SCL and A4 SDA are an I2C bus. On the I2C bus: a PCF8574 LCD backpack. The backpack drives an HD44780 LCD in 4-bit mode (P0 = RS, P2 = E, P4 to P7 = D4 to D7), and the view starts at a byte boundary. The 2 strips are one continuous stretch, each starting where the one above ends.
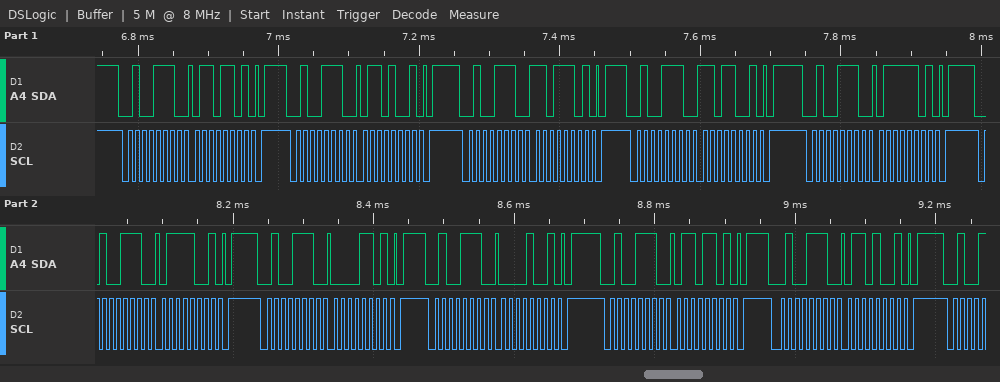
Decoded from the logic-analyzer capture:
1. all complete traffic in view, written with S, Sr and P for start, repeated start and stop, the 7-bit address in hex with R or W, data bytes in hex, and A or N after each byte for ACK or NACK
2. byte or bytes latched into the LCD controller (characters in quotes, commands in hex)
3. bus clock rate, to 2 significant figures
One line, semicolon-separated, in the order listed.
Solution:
S 27W A 6D A P S 27W A 69 A P S 27W A DD A P S 27W A D9 A P S 27W A 7D A P S 27W A 79 A P S 27W A 0D A P S 27W A 09 A P S 27W A 6D A P S 27W A 69 A P; 'm' 'p'; 100 kHz
